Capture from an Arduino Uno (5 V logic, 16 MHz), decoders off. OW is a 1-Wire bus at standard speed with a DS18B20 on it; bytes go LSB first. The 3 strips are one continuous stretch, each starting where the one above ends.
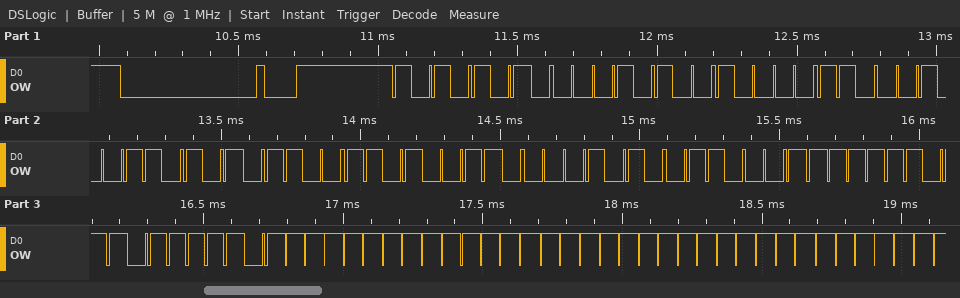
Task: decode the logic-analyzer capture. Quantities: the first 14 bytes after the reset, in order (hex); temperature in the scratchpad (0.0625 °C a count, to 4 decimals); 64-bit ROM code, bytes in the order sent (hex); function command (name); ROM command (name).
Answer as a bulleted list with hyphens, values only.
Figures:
- 55 28 61 64 35 CB 50 C6 DF BE FF FF FF FF
- -0.0625 °C
- 28 61 64 35 CB 50 C6 DF
- Read Scratchpad
- Match ROM
